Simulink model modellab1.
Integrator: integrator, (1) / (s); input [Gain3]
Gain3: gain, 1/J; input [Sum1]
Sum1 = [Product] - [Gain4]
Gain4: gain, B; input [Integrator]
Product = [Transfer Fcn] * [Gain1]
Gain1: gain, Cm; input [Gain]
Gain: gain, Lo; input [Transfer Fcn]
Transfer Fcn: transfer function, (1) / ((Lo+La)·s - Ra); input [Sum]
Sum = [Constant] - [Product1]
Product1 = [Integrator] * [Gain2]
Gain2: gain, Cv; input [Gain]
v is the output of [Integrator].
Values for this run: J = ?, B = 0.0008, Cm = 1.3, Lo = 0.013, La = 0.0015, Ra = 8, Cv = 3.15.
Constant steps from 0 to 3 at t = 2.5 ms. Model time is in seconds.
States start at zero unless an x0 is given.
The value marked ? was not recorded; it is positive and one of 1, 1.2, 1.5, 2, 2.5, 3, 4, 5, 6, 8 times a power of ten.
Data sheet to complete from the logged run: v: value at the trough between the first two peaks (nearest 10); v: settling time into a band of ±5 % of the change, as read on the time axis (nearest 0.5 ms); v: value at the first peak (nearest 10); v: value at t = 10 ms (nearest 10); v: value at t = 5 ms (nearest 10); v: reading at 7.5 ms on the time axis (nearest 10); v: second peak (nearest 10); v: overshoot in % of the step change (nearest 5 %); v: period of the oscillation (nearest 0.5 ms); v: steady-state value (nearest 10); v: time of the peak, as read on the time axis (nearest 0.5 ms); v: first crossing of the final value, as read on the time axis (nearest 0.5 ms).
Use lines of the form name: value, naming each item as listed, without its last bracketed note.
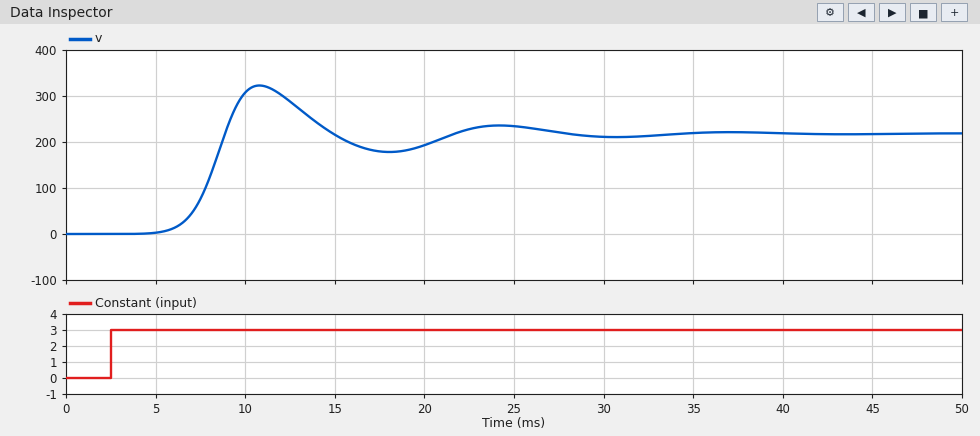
v: value at the trough between the first two peaks: 180
v: settling time into a band of ±5 % of the change, as read on the time axis: 26.0 ms
v: value at the first peak: 320
v: value at t = 10 ms: 310
v: value at t = 5 ms: 0
v: reading at 7.5 ms on the time axis: 80
v: second peak: 240
v: overshoot in % of the step change: 50 %
v: period of the oscillation: 13.5 ms
v: steady-state value: 220
v: time of the peak, as read on the time axis: 11.0 ms
v: first crossing of the final value, as read on the time axis: 9.0 ms
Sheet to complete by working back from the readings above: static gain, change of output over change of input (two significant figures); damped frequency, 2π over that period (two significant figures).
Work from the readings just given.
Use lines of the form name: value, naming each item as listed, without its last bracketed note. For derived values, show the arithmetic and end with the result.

static gain, change of output over change of input: (220 - 0) / (3 - 0) = 73
damped frequency, 2π over that period: 2π / 13.5 = 0.47 rad/ms
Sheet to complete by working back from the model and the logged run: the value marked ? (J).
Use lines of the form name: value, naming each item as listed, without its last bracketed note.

the value marked ?: 4e-06
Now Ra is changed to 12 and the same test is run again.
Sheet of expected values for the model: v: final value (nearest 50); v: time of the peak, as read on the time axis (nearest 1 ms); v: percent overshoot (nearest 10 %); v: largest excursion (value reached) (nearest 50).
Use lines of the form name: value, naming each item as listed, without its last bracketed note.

v: final value: 300
v: time of the peak, as read on the time axis: 9 ms
v: percent overshoot: 60 %
v: largest excursion (value reached): 500
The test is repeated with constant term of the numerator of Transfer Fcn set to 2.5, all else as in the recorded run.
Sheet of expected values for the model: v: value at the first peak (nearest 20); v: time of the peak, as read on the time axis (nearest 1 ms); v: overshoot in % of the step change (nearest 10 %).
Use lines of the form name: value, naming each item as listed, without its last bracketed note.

v: value at the first peak: 160
v: time of the peak, as read on the time axis: 8 ms
v: overshoot in % of the step change: 40 %
